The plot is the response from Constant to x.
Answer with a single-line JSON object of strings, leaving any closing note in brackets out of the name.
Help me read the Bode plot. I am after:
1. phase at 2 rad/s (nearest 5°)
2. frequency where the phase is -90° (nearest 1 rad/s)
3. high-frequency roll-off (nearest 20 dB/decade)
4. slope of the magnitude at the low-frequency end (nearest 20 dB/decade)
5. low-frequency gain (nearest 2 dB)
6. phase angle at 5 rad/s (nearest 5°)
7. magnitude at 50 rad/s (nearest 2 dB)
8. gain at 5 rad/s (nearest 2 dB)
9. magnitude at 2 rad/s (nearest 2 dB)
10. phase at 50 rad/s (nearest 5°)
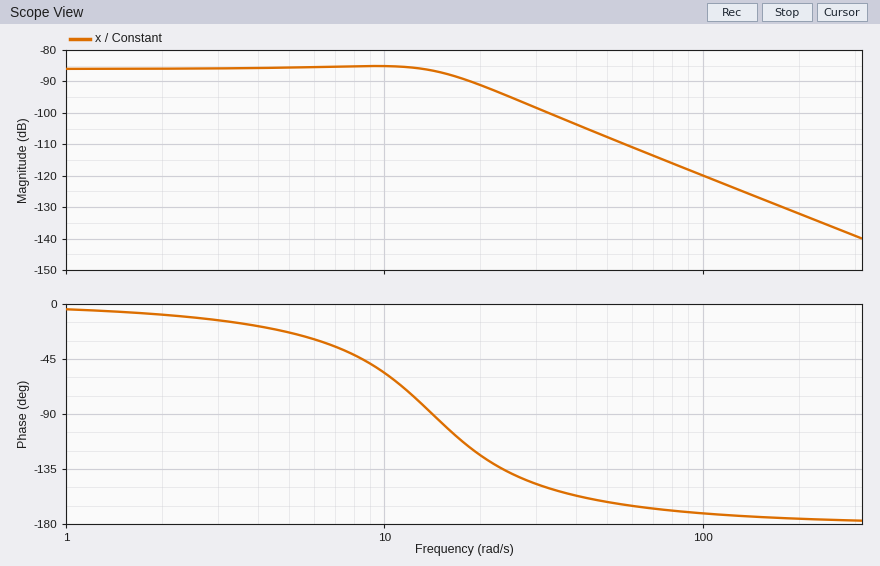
{"phase at 2 rad/s": "-10°", "frequency where the phase is -90°": "14 rad/s", "high-frequency roll-off": "-40 dB/decade", "slope of the magnitude at the low-frequency end": "0 dB/decade", "low-frequency gain": "-86 dB", "phase angle at 5 rad/s": "-25°", "magnitude at 50 rad/s": "-108 dB", "gain at 5 rad/s": "-86 dB", "magnitude at 2 rad/s": "-86 dB", "phase at 50 rad/s": "-160°"}
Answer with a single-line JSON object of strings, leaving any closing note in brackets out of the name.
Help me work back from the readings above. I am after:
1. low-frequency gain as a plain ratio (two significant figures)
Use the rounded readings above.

{"low-frequency gain as a plain ratio": "0.000050"}
